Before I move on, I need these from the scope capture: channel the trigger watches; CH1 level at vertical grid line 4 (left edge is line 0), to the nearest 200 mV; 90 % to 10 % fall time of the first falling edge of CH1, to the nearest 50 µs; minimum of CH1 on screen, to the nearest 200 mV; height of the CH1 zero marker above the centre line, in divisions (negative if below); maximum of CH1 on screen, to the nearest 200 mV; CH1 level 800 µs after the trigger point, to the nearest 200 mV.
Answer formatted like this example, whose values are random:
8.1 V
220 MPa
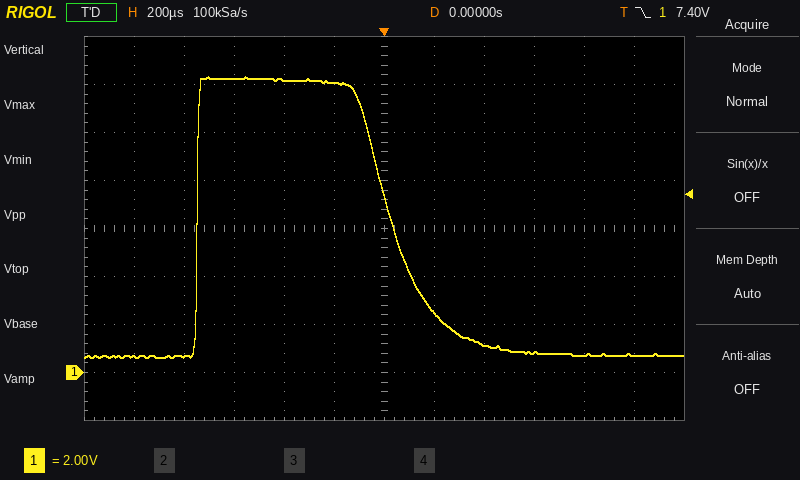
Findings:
CH1
12.2 V
350 µs
600 mV
-3.0 div
12.4 V
800 mV
